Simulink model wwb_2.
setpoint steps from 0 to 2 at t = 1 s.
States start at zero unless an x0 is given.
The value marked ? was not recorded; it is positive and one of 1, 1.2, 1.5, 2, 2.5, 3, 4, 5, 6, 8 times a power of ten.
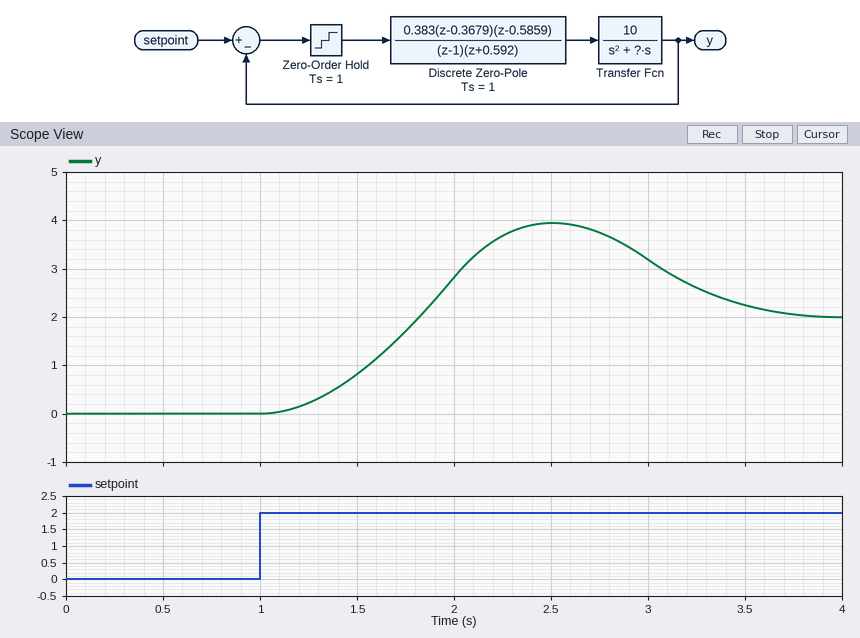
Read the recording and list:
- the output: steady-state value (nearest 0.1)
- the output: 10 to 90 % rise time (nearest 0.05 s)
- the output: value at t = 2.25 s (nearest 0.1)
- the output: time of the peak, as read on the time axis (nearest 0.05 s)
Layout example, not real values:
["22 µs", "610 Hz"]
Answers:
["2.0", "0.55 s", "3.7", "2.50 s"]
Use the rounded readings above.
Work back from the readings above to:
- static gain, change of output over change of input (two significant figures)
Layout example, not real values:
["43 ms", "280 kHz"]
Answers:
["1.0"]
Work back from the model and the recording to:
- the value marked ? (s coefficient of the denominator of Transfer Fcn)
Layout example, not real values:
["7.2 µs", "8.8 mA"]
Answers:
["1"]
